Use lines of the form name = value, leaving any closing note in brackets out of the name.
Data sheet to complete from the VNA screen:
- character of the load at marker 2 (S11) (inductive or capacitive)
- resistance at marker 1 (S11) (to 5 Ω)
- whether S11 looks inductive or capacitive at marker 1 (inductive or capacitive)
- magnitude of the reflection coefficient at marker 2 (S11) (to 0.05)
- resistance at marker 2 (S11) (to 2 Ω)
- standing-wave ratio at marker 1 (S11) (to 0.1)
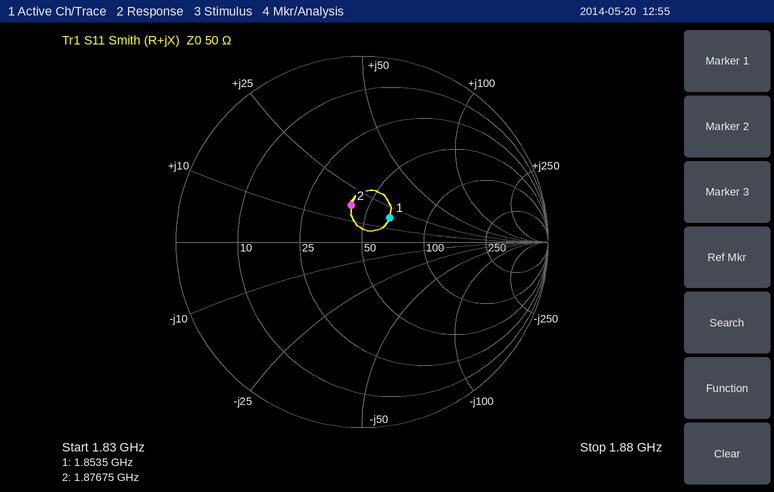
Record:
character of the load at marker 2 (S11) = inductive
resistance at marker 1 (S11) = 65 Ω
whether S11 looks inductive or capacitive at marker 1 = inductive
magnitude of the reflection coefficient at marker 2 (S11) = 0.20
resistance at marker 2 (S11) = 42 Ω
standing-wave ratio at marker 1 (S11) = 1.5
